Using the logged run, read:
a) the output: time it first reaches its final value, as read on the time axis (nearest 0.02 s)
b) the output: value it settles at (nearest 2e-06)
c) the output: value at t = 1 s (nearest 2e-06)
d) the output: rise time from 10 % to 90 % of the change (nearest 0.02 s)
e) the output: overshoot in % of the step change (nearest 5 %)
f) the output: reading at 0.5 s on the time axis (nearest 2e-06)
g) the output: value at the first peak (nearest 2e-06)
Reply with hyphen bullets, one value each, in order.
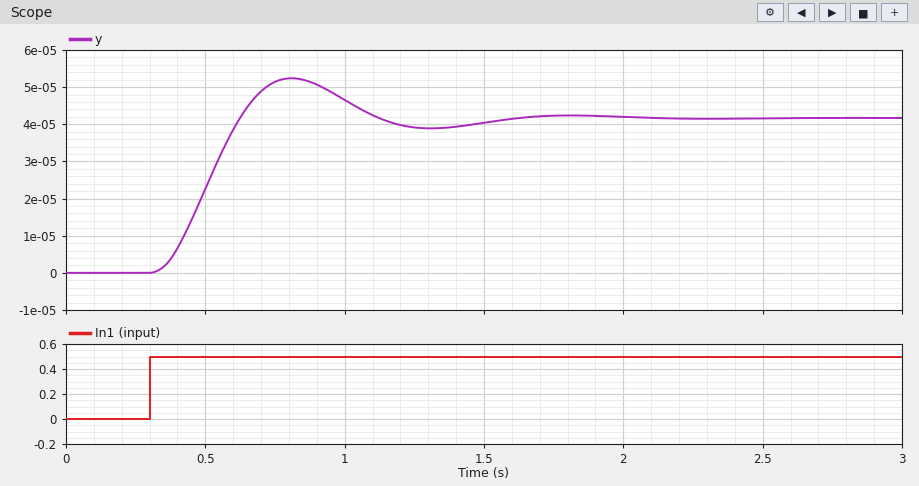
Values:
- 0.62 s
- 0.000042
- 0.000046
- 0.22 s
- 25 %
- 0.000022
- 0.000052
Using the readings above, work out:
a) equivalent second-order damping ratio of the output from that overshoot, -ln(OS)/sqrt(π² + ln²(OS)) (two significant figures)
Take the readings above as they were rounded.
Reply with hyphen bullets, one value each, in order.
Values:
- 0.40
